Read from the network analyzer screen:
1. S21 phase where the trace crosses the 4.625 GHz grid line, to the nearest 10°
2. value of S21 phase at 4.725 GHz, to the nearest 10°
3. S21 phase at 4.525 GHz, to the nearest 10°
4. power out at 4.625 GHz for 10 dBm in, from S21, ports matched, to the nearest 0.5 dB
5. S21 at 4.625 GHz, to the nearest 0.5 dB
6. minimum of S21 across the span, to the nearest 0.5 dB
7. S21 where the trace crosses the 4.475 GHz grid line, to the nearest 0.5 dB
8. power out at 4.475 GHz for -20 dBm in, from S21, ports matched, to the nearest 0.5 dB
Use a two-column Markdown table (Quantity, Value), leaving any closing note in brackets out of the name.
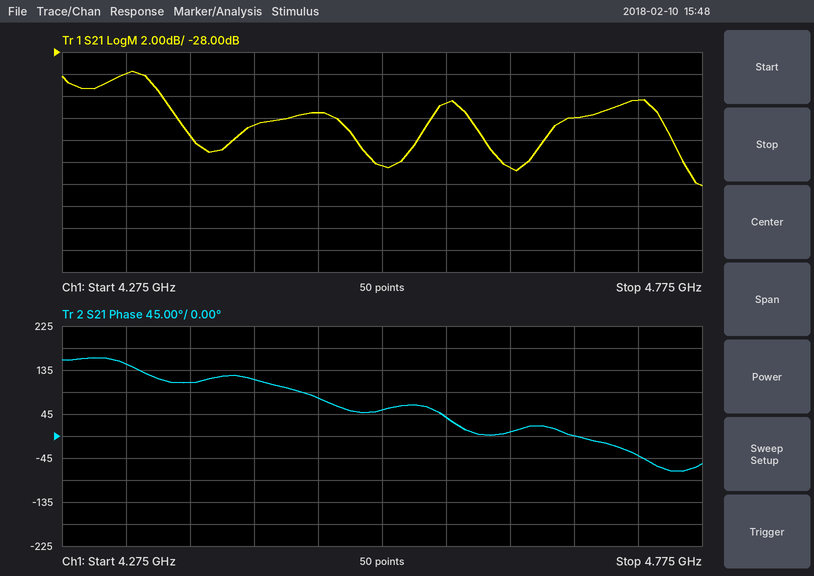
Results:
| Quantity | Value |
|---|---|
| S21 phase where the trace crosses the 4.625 GHz grid line, to the nearest 10° | 10° |
| value of S21 phase at 4.725 GHz, to the nearest 10° | -40° |
| S21 phase at 4.525 GHz, to the nearest 10° | 50° |
| power out at 4.625 GHz for 10 dBm in, from S21, ports matched, to the nearest 0.5 dB | -28.5 dBm |
| S21 at 4.625 GHz, to the nearest 0.5 dB | -38.5 dB |
| minimum of S21 across the span, to the nearest 0.5 dB | -40.0 dB |
| S21 where the trace crosses the 4.475 GHz grid line, to the nearest 0.5 dB | -33.5 dB |
| power out at 4.475 GHz for -20 dBm in, from S21, ports matched, to the nearest 0.5 dB | -53.5 dBm |
